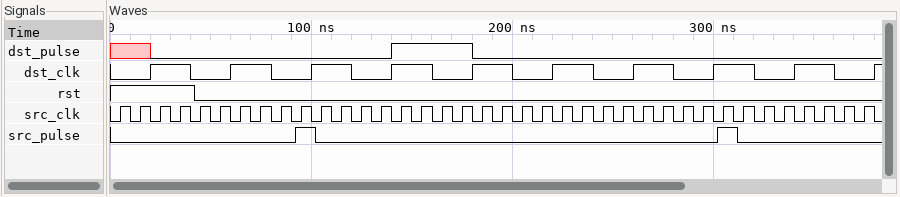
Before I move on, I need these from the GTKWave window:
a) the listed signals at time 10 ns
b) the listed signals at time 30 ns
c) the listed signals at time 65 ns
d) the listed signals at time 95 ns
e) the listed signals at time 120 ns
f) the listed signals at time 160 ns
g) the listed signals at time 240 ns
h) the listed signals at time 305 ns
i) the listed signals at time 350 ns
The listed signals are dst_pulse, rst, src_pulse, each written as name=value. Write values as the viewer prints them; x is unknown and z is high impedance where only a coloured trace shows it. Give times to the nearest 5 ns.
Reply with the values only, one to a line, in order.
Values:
dst_pulse=x, rst=1, src_pulse=0
dst_pulse=0, rst=1, src_pulse=0
dst_pulse=0, rst=0, src_pulse=0
dst_pulse=0, rst=0, src_pulse=1
dst_pulse=0, rst=0, src_pulse=0
dst_pulse=1, rst=0, src_pulse=0
dst_pulse=0, rst=0, src_pulse=0
dst_pulse=0, rst=0, src_pulse=1
dst_pulse=0, rst=0, src_pulse=0
